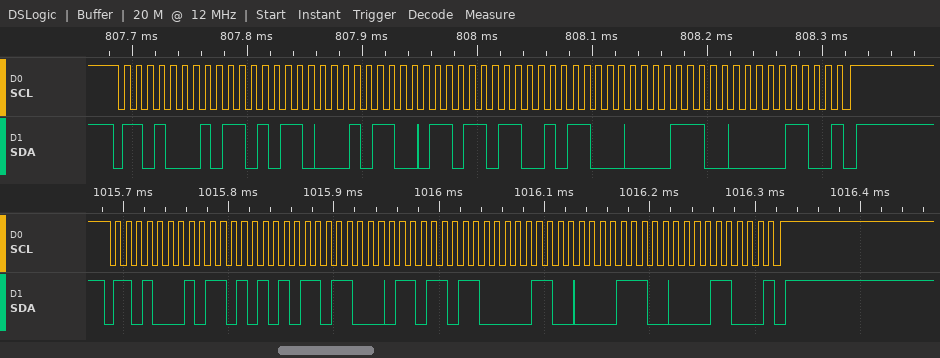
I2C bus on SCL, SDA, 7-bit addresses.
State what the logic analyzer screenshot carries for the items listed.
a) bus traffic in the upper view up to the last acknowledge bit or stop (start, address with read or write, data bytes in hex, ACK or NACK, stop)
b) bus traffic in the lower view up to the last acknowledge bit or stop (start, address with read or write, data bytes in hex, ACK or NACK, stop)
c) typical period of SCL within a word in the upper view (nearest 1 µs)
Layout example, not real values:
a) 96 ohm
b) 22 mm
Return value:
a) start, address 68 read ACK, D6 ACK, 2C ACK, DB ACK, 58 ACK, 1C ACK, 0C NACK, stop
b) start, address 68 read ACK, D5 ACK, D8 ACK, DB ACK, 0C ACK, 1C ACK, 18 NACK, stop
c) 10 µs
